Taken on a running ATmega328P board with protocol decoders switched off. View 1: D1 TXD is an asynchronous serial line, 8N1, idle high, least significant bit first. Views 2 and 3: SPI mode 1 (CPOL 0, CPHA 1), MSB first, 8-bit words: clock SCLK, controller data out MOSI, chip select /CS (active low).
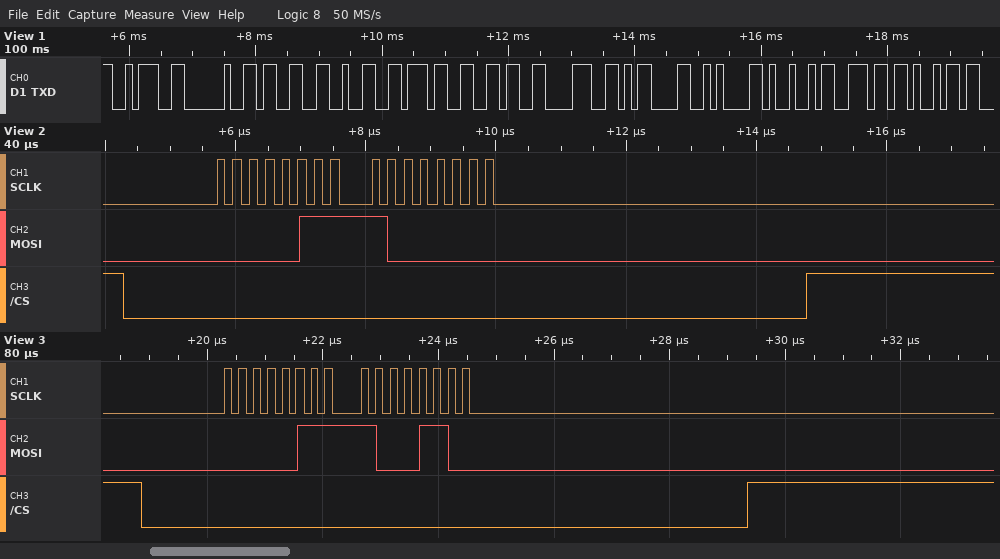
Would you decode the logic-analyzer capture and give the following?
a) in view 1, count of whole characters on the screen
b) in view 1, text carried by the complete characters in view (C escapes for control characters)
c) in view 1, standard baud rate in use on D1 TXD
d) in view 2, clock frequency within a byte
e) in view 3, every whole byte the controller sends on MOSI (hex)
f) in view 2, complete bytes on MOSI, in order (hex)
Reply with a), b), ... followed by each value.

a) 12
b) ": 32768\r\nIni"
c) 9600 baud
d) 4 MHz
e) 07 8C
f) 07 80
